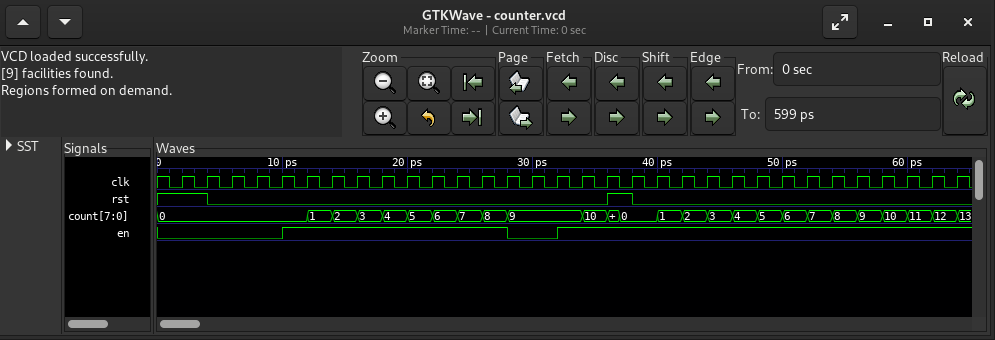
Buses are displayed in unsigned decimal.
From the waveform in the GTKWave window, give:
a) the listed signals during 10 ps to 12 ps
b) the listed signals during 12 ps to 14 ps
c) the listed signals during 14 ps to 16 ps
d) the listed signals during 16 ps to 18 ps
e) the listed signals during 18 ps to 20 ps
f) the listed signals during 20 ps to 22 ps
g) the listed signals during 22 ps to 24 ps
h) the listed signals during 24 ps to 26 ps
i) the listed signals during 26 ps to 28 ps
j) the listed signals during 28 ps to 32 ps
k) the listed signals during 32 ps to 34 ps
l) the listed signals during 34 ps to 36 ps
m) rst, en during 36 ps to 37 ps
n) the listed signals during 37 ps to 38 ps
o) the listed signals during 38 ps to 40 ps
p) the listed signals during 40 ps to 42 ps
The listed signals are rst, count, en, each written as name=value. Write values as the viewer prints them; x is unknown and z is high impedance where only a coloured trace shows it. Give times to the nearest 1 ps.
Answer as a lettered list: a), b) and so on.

a) rst=0, count=0, en=1
b) rst=0, count=1, en=1
c) rst=0, count=2, en=1
d) rst=0, count=3, en=1
e) rst=0, count=4, en=1
f) rst=0, count=5, en=1
g) rst=0, count=6, en=1
h) rst=0, count=7, en=1
i) rst=0, count=8, en=1
j) rst=0, count=9, en=0
k) rst=0, count=9, en=1
l) rst=0, count=10, en=1
m) rst=1, en=1
n) rst=1, count=0, en=1
o) rst=0, count=0, en=1
p) rst=0, count=1, en=1
